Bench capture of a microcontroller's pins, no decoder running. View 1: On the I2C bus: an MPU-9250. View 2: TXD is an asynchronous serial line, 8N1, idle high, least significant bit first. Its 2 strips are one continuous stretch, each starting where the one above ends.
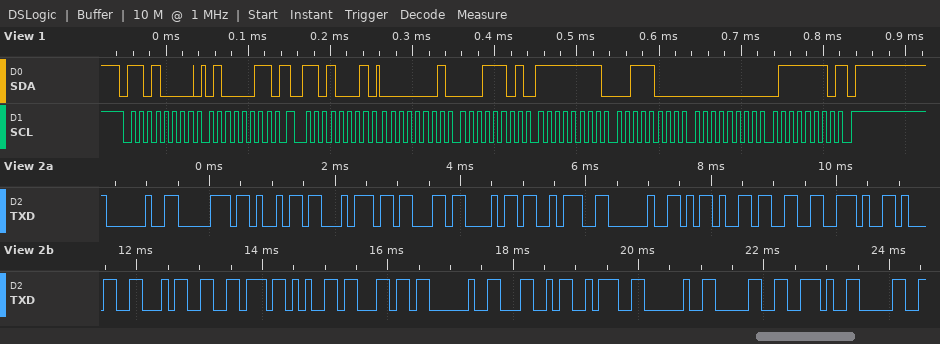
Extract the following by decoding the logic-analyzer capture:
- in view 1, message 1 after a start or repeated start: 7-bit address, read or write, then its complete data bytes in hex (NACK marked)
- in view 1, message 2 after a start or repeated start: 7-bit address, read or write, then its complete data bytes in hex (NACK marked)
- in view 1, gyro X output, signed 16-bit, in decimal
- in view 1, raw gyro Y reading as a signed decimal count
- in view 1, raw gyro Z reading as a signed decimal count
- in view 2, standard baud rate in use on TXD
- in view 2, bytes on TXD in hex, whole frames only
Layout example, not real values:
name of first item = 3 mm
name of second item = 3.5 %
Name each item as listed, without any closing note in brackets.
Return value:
in view 1, message 1 after a start or repeated start: 7-bit address, read or write, then its complete data bytes in hex = 0x68 write: 43
in view 1, message 2 after a start or repeated start: 7-bit address, read or write, then its complete data bytes in hex = 0x68 read: 01 1D FF 38 00 7E NACK
in view 1, gyro X output, signed 16-bit, in decimal = 285
in view 1, raw gyro Y reading as a signed decimal count = -200
in view 1, raw gyro Z reading as a signed decimal count = 126
in view 2, standard baud rate in use on TXD = 9600 baud
in view 2, bytes on TXD in hex, whole frames only = 20 70 69 74 63 68 3A 20 2D 33 2E 31 34 76 65 6C 20 4C 3A 20 30 2E 30
